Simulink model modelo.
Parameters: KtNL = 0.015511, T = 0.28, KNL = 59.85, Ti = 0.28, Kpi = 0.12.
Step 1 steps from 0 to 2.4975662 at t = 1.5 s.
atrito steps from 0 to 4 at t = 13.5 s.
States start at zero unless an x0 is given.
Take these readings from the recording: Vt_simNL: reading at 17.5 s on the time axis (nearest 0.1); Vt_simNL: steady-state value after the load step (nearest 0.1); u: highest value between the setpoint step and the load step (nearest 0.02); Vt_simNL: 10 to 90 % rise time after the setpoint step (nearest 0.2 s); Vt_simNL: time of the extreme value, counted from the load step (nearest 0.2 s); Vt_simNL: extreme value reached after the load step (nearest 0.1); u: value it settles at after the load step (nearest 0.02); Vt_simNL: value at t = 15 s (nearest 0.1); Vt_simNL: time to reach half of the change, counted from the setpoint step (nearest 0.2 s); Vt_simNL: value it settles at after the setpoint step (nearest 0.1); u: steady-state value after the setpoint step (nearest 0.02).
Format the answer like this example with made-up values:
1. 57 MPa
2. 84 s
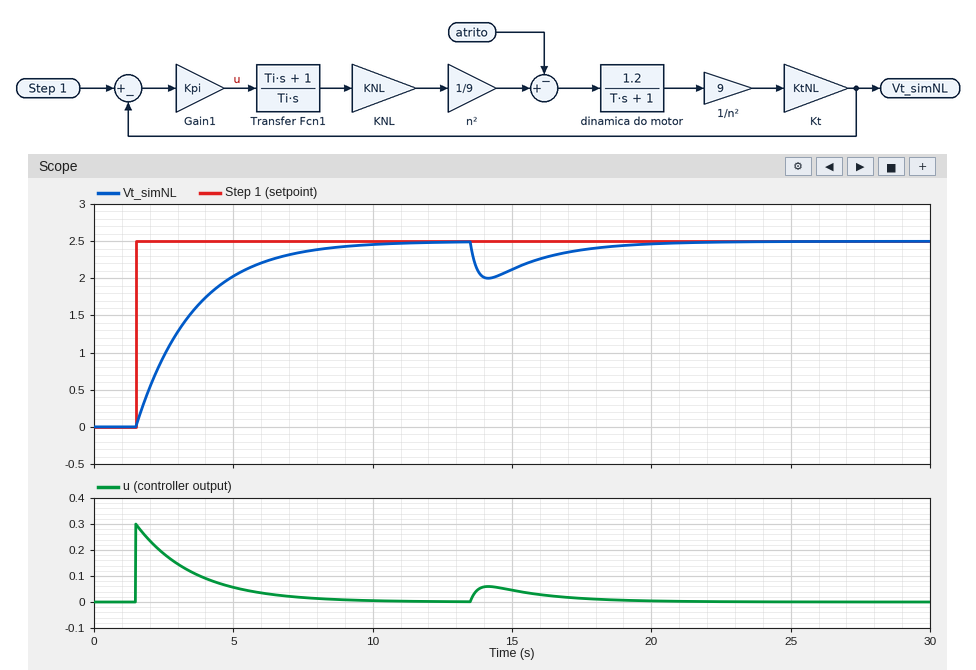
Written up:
1. 2.4
2. 2.5
3. 0.30
4. 4.6 s
5. 0.6 s
6. 2.0
7. 0.00
8. 2.1
9. 1.4 s
10. 2.5
11. 0.00
